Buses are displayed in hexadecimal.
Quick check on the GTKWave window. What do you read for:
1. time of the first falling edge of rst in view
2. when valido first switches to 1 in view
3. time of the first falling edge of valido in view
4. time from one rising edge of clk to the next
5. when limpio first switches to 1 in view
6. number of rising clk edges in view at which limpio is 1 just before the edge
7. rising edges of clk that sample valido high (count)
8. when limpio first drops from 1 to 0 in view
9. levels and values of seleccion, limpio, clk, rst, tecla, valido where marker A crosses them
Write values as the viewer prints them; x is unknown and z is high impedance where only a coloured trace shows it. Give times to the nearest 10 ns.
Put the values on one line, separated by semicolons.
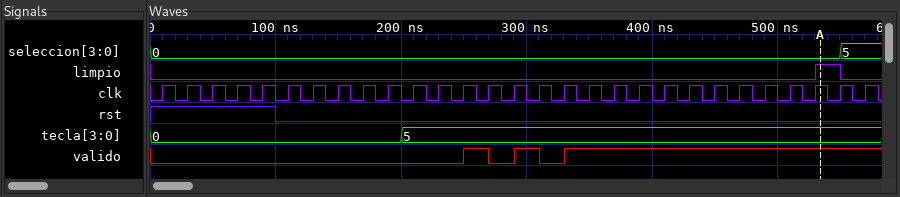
100 ns; 250 ns; 270 ns; 20 ns; 530 ns; 1; 14; 550 ns; seleccion=0, limpio=1, clk=1, rst=0, tecla=5, valido=1
